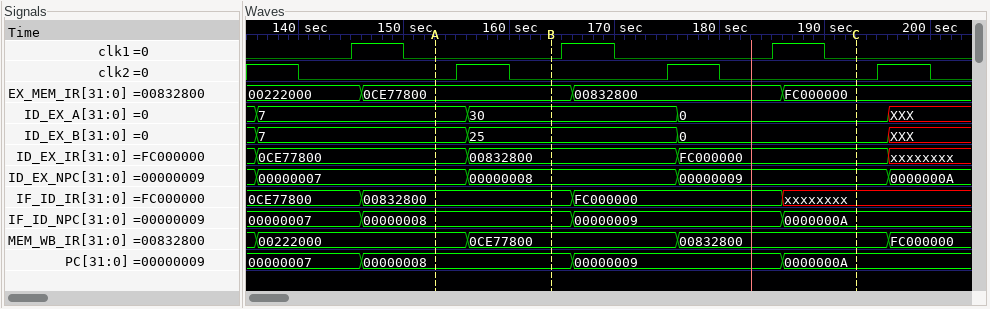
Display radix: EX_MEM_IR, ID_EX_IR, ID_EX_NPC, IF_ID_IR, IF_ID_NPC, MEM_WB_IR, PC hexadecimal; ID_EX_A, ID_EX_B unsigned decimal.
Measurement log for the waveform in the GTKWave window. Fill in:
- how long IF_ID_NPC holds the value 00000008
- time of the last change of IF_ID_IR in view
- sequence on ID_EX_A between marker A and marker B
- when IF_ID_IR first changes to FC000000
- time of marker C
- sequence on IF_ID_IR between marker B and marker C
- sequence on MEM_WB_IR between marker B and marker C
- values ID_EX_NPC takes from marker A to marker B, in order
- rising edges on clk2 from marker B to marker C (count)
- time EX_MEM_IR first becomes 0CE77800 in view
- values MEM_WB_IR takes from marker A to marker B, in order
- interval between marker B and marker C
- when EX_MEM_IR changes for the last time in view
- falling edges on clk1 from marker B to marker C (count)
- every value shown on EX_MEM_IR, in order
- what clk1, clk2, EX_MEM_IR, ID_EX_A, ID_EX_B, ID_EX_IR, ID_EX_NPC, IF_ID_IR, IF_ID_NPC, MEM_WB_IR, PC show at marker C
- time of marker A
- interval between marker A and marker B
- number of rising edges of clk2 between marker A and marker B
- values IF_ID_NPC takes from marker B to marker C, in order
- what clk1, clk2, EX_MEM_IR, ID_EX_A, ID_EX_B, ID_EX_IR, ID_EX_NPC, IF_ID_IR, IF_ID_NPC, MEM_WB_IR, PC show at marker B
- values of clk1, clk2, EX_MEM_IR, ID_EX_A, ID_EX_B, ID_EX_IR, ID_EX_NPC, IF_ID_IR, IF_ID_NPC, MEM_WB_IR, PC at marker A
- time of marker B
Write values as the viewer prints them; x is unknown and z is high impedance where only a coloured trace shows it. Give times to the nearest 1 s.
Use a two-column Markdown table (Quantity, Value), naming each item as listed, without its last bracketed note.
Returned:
| Quantity | Value |
|---|---|
| how long IF_ID_NPC holds the value 00000008 | 20 s |
| time of the last change of IF_ID_IR in view | 186 s |
| sequence on ID_EX_A between marker A and marker B | 7, 30 |
| when IF_ID_IR first changes to FC000000 | 166 s |
| time of marker C | 193 s |
| sequence on IF_ID_IR between marker B and marker C | 00832800, FC000000, xxxxxxxx |
| sequence on MEM_WB_IR between marker B and marker C | 0CE77800, 00832800 |
| values ID_EX_NPC takes from marker A to marker B, in order | 00000007, 00000008 |
| rising edges on clk2 from marker B to marker C | 1 |
| time EX_MEM_IR first becomes 0CE77800 in view | 146 s |
| values MEM_WB_IR takes from marker A to marker B, in order | 00222000, 0CE77800 |
| interval between marker B and marker C | 29 s |
| when EX_MEM_IR changes for the last time in view | 186 s |
| falling edges on clk1 from marker B to marker C | 2 |
| every value shown on EX_MEM_IR, in order | 00222000, 0CE77800, 00832800, FC000000 |
| what clk1, clk2, EX_MEM_IR, ID_EX_A, ID_EX_B, ID_EX_IR, ID_EX_NPC, IF_ID_IR, IF_ID_NPC, MEM_WB_IR, PC show at marker C | clk1=0, clk2=0, EX_MEM_IR=FC000000, ID_EX_A=0, ID_EX_B=0, ID_EX_IR=FC000000, ID_EX_NPC=00000009, IF_ID_IR=xxxxxxxx, IF_ID_NPC=0000000A, MEM_WB_IR=00832800, PC=0000000A |
| time of marker A | 153 s |
| interval between marker A and marker B | 11 s |
| number of rising edges of clk2 between marker A and marker B | 1 |
| values IF_ID_NPC takes from marker B to marker C, in order | 00000008, 00000009, 0000000A |
| what clk1, clk2, EX_MEM_IR, ID_EX_A, ID_EX_B, ID_EX_IR, ID_EX_NPC, IF_ID_IR, IF_ID_NPC, MEM_WB_IR, PC show at marker B | clk1=0, clk2=0, EX_MEM_IR=0CE77800, ID_EX_A=30, ID_EX_B=25, ID_EX_IR=00832800, ID_EX_NPC=00000008, IF_ID_IR=00832800, IF_ID_NPC=00000008, MEM_WB_IR=0CE77800, PC=00000008 |
| values of clk1, clk2, EX_MEM_IR, ID_EX_A, ID_EX_B, ID_EX_IR, ID_EX_NPC, IF_ID_IR, IF_ID_NPC, MEM_WB_IR, PC at marker A | clk1=0, clk2=0, EX_MEM_IR=0CE77800, ID_EX_A=7, ID_EX_B=7, ID_EX_IR=0CE77800, ID_EX_NPC=00000007, IF_ID_IR=00832800, IF_ID_NPC=00000008, MEM_WB_IR=00222000, PC=00000008 |
| time of marker B | 164 s |
